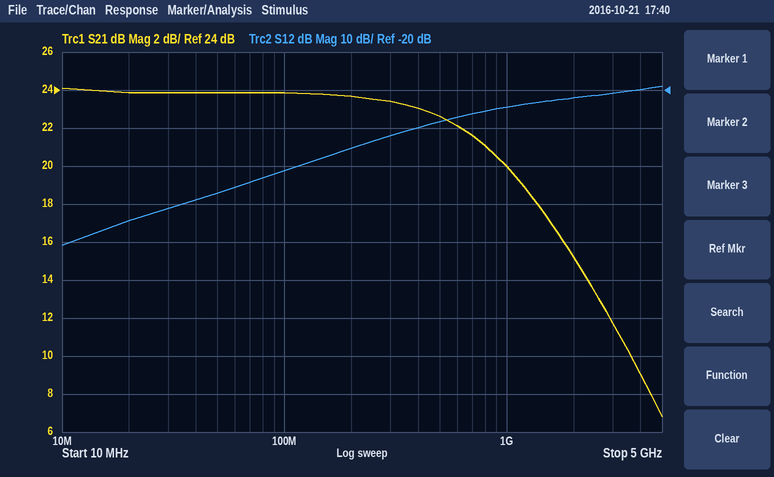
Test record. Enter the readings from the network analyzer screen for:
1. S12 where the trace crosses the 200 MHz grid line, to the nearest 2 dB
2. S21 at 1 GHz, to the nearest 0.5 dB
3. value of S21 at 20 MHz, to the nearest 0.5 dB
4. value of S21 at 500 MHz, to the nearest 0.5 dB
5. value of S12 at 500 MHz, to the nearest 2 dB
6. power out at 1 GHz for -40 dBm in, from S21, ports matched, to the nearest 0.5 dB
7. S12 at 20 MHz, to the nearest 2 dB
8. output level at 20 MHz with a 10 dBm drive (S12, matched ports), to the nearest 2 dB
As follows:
-36 dB
20.0 dB
24.0 dB
22.5 dB
-28 dB
-20.0 dBm
-54 dB
-44 dBm
